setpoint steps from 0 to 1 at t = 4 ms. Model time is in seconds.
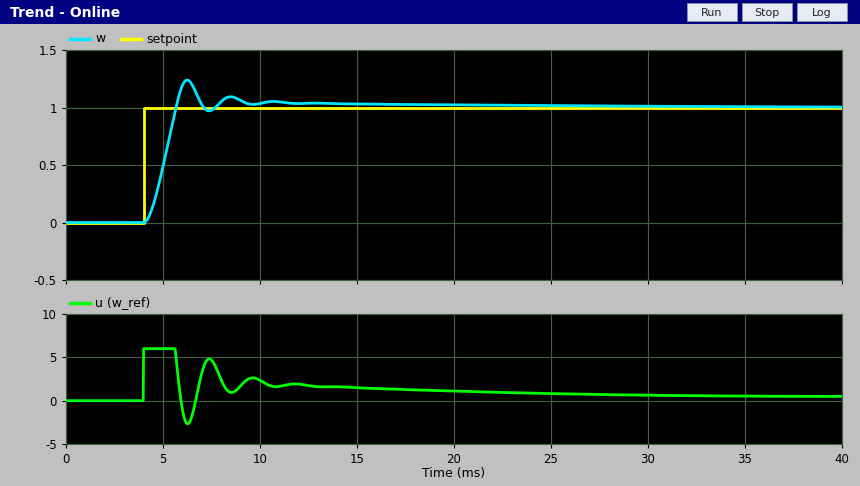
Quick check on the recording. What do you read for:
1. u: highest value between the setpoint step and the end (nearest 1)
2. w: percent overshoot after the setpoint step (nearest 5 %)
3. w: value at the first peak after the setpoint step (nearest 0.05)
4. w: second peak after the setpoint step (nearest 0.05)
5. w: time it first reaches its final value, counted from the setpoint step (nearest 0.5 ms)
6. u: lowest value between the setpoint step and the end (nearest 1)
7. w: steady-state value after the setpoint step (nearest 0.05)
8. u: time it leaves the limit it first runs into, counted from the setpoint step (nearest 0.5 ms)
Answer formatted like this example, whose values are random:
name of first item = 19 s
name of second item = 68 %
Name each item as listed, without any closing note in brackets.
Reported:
u: highest value between the setpoint step and the end = 6
w: percent overshoot after the setpoint step = 25 %
w: value at the first peak after the setpoint step = 1.25
w: second peak after the setpoint step = 1.10
w: time it first reaches its final value, counted from the setpoint step = 1.5 ms
u: lowest value between the setpoint step and the end = -3
w: steady-state value after the setpoint step = 1.00
u: time it leaves the limit it first runs into, counted from the setpoint step = 1.5 ms
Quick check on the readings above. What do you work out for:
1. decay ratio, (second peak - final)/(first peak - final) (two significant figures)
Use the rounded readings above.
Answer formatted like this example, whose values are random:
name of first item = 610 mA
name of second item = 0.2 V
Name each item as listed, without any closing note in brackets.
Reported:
decay ratio, (second peak - final)/(first peak - final) = 0.40
